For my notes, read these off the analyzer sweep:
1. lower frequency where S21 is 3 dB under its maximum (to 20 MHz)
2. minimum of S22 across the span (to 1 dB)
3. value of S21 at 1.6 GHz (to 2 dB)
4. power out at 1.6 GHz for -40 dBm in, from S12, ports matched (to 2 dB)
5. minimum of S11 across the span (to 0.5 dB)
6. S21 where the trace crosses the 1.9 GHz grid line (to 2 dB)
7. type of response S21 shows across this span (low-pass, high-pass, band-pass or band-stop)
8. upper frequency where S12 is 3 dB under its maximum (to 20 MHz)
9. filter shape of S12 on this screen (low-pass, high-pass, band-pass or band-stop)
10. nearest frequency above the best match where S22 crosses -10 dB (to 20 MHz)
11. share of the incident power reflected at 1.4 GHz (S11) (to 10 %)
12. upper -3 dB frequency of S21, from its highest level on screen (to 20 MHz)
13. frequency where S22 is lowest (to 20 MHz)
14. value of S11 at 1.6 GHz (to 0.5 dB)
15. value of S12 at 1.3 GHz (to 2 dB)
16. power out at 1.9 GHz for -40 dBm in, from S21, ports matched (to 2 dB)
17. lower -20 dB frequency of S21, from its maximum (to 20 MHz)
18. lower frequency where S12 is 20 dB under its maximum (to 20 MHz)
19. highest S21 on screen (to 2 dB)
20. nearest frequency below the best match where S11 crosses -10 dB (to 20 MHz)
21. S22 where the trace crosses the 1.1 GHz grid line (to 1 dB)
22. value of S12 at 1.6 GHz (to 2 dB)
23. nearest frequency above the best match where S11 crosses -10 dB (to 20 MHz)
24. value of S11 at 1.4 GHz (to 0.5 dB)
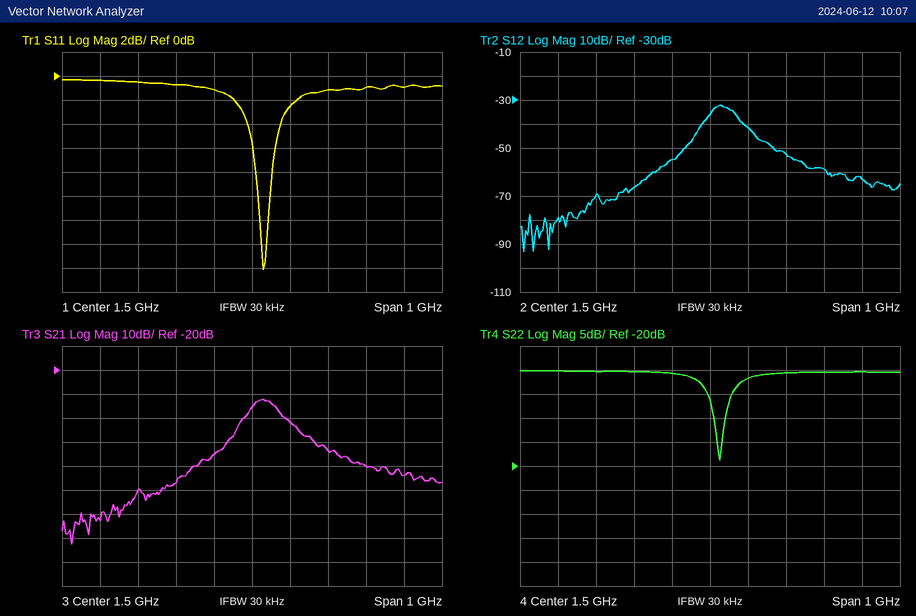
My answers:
1.50 GHz
-19 dB
-42 dB
-82 dBm
-16.0 dB
-64 dB
band-pass
1.56 GHz
band-pass
1.54 GHz
80 %
1.56 GHz
1.52 GHz
-2.5 dB
-66 dB
-104 dBm
1.42 GHz
1.42 GHz
-32 dB
1.52 GHz
0 dB
-42 dB
1.54 GHz
-1.0 dB
